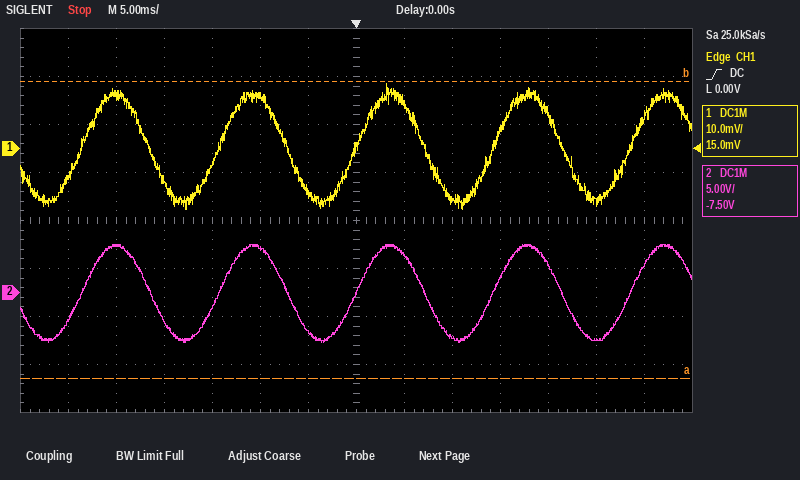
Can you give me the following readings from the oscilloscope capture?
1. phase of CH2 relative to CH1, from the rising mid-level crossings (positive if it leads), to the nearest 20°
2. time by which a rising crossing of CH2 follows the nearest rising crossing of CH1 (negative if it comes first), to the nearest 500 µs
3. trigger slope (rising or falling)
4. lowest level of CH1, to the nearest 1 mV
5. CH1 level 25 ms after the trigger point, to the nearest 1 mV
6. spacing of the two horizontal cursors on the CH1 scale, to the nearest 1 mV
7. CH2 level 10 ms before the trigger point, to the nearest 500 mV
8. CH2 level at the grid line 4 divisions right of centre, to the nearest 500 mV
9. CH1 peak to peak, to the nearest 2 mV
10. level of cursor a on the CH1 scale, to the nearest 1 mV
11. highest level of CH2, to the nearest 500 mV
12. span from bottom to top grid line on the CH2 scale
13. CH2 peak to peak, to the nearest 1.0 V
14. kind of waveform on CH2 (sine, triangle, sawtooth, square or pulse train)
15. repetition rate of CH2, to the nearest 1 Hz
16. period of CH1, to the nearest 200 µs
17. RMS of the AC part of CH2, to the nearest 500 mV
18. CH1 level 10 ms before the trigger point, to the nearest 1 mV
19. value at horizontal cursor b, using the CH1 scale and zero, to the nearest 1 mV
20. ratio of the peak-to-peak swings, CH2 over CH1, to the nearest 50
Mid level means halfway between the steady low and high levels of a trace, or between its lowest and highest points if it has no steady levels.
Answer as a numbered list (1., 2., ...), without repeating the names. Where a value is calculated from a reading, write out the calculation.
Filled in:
1. −360° × (0.0 ms) / 14.4 ms ≈ 0°
2. 0.0 ms
3. rising
4. -13 mV
5. -11 mV
6. 62 mV
7. 4.5 V
8. 3.0 V
9. 26 mV
10. -48 mV
11. 5.0 V
12. 40 V
13. 10.0 V
14. sine
15. 70 Hz
16. 14.4 ms
17. 10.0 V / (2√2) ≈ 3.5 V
18. 11 mV
19. 14 mV
20. 10.0 V / 26 mV ≈ 385, so 400 to the nearest 50
